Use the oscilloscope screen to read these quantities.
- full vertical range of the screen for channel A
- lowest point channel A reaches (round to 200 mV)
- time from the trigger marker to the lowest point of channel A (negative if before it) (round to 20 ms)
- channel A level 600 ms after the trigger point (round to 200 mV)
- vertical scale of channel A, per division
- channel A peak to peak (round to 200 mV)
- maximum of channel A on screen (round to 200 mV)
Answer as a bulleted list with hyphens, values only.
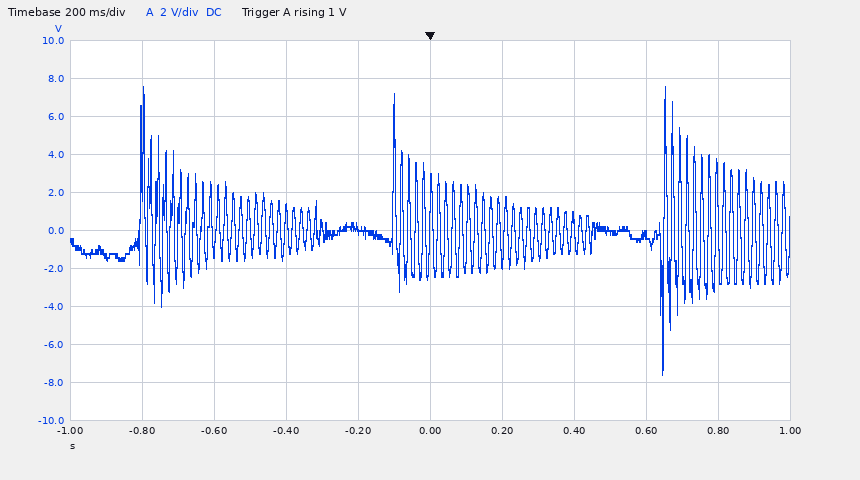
- 20 V
- -7.6 V
- +640 ms
- -200 mV
- 2 V
- 15.2 V
- 7.6 V
